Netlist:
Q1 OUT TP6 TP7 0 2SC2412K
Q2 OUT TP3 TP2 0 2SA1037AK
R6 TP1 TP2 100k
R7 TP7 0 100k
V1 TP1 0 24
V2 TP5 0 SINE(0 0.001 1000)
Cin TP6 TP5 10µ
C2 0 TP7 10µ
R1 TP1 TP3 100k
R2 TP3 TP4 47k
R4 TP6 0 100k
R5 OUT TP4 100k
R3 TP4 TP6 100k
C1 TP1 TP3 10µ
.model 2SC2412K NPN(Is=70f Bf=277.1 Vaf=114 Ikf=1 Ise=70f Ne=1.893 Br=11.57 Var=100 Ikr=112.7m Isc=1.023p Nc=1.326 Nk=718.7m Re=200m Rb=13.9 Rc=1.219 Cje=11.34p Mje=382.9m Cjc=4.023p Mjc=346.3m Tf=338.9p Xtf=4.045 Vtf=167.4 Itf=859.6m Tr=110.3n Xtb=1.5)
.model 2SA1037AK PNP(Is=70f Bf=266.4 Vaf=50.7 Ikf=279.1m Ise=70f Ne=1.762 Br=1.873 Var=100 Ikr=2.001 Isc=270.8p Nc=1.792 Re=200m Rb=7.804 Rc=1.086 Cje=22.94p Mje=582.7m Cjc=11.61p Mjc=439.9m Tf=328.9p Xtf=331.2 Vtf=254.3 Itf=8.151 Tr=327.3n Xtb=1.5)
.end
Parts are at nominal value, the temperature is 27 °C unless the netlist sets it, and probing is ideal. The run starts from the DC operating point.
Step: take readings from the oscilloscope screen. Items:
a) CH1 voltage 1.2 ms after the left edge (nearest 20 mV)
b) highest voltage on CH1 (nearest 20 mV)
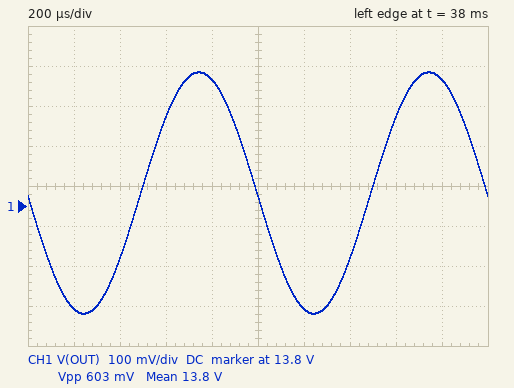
13.54 V
14.14 V
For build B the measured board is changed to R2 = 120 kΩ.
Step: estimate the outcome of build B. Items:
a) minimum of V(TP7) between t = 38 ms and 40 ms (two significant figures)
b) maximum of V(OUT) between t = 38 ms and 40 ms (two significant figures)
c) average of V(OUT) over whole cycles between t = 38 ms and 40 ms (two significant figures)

5.2 V
12 V
11 V
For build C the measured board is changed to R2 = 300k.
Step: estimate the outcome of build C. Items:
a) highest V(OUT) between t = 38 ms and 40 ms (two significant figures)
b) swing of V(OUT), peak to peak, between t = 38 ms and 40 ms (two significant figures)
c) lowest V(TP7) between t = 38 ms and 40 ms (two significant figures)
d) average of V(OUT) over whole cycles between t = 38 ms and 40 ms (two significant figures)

8.2 V
440 mV
3.5 V
8.0 V
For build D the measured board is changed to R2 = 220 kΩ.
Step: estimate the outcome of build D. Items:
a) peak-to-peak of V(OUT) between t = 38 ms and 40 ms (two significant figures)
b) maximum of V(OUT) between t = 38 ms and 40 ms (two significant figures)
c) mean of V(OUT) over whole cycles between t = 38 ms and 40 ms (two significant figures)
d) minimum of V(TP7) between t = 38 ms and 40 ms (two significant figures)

500 mV
9.5 V
9.2 V
4.1 V
